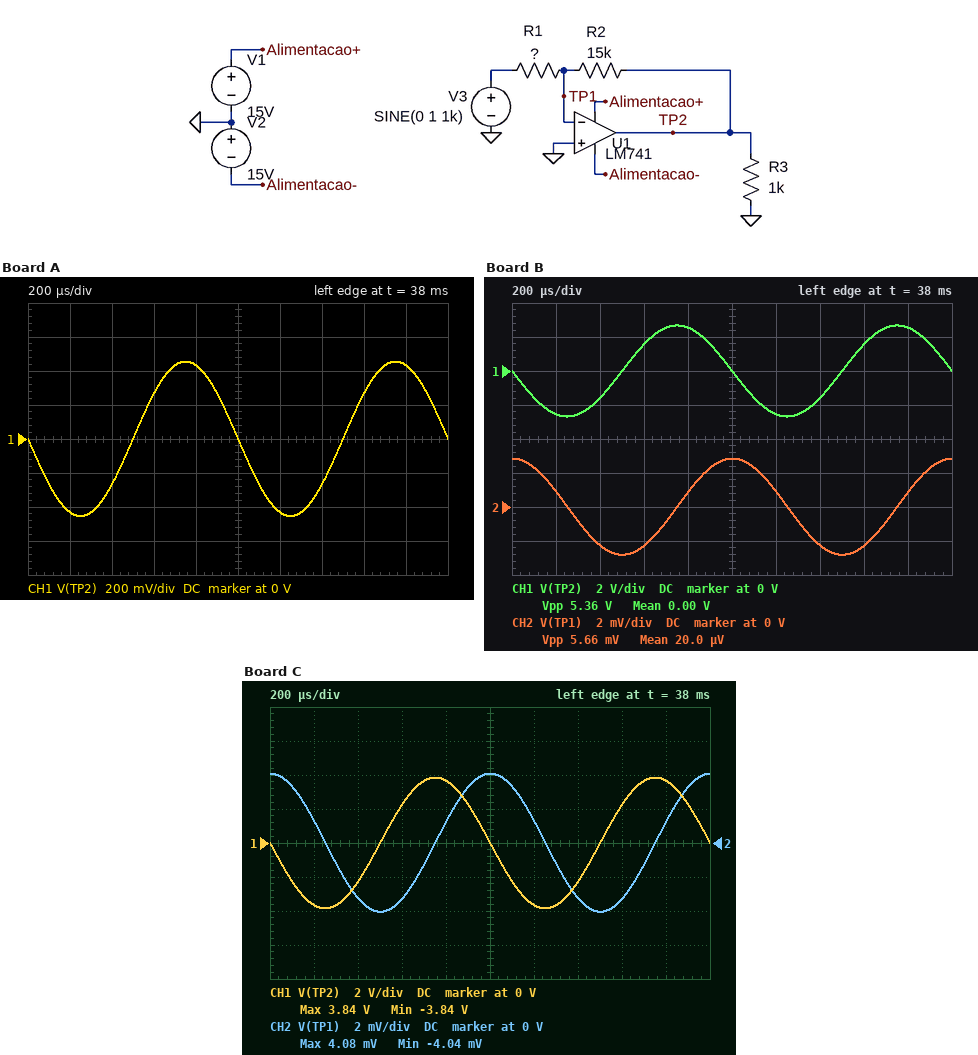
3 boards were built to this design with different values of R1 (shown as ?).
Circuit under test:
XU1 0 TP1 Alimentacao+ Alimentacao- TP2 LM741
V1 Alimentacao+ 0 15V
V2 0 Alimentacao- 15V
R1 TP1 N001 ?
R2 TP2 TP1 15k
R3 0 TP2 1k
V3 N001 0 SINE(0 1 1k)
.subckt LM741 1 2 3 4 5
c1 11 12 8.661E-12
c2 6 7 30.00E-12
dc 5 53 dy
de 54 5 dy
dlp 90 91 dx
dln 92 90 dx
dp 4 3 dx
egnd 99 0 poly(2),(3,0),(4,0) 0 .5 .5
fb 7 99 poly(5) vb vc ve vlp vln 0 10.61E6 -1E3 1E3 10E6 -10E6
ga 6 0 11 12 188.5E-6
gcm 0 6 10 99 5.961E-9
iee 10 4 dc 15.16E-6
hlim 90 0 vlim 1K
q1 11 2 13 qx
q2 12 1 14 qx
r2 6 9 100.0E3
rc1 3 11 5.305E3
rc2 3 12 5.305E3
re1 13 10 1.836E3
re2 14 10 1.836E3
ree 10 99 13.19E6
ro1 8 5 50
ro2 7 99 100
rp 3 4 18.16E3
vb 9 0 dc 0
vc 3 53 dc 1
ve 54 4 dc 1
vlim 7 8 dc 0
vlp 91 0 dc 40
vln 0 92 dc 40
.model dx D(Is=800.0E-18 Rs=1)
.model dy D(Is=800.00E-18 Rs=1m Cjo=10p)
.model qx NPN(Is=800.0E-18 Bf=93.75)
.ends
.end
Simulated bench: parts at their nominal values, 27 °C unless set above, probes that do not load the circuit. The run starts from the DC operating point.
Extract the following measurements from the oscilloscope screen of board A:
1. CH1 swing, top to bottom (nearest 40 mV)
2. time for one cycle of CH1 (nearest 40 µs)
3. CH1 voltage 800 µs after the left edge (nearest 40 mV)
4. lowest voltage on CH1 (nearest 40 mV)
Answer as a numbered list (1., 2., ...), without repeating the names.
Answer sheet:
1. 920 mV
2. 1.00 ms
3. 440 mV
4. -440 mV
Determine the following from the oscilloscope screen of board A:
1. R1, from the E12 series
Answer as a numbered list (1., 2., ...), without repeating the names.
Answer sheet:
1. 33 kΩ
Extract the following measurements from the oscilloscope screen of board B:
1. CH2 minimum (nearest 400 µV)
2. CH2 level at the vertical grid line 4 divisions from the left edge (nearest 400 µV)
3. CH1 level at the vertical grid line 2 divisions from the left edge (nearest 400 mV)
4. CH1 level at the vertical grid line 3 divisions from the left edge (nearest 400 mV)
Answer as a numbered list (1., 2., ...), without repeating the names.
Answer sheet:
1. -2.8 mV
2. 800 µV
3. -1.6 V
4. 1.6 V
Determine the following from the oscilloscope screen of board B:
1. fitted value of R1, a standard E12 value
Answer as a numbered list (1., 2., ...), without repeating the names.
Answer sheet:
1. 5.6 kΩ
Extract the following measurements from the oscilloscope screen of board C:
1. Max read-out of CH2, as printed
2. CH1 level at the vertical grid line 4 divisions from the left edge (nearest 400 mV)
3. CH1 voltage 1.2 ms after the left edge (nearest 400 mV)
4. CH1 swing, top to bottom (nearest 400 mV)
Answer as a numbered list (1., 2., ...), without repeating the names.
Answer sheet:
1. 4.08 mV
2. 3.6 V
3. -3.6 V
4. 7.6 V
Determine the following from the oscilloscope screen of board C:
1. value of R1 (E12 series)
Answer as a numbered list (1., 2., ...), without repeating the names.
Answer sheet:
1. 3.9 kΩ
